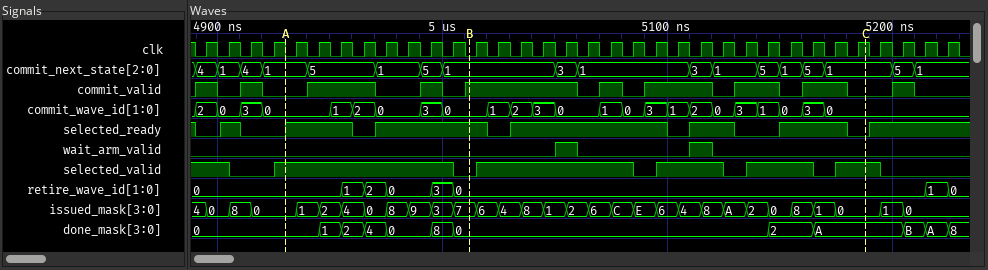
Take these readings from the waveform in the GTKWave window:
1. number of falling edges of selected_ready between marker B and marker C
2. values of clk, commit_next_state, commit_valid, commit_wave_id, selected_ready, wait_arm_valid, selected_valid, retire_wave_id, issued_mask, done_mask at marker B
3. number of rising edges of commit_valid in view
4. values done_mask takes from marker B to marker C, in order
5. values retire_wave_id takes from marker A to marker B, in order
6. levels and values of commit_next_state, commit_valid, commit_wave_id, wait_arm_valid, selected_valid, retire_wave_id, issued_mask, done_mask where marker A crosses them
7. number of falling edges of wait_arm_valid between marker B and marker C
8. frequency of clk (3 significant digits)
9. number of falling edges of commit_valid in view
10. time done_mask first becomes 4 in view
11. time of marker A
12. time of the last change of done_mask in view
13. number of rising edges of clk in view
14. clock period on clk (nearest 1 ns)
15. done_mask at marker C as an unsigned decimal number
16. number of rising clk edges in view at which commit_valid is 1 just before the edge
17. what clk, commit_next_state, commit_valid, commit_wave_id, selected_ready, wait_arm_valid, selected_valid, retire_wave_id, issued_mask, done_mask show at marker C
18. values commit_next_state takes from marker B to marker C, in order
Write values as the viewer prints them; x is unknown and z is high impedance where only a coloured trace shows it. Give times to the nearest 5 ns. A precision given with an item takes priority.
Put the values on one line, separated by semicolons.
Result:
4; clk=0, commit_next_state=1, commit_valid=1, commit_wave_id=0, selected_ready=1, wait_arm_valid=0, selected_valid=0, retire_wave_id=0, issued_mask=7, done_mask=0; 10; 0, 2, A; 0, 1, 2, 0, 3, 0; commit_next_state=1, commit_valid=0, commit_wave_id=0, wait_arm_valid=0, selected_valid=1, retire_wave_id=0, issued_mask=0, done_mask=0; 2; 100 MHz; 10; 4965 ns; 4930 ns; 5225 ns; 34; 10 ns; 10; 20; clk=1, commit_next_state=1, commit_valid=0, commit_wave_id=0, selected_ready=0, wait_arm_valid=0, selected_valid=1, retire_wave_id=0, issued_mask=0, done_mask=A; 1, 3, 1, 3, 1, 5, 1, 5, 1
